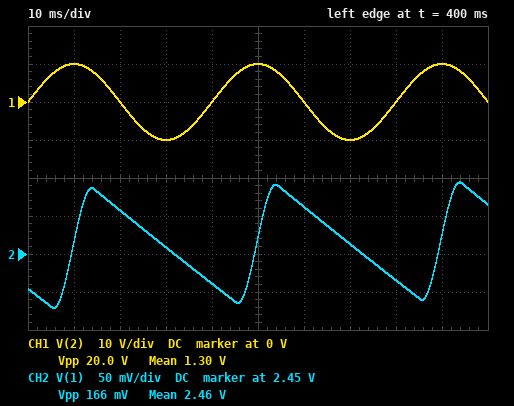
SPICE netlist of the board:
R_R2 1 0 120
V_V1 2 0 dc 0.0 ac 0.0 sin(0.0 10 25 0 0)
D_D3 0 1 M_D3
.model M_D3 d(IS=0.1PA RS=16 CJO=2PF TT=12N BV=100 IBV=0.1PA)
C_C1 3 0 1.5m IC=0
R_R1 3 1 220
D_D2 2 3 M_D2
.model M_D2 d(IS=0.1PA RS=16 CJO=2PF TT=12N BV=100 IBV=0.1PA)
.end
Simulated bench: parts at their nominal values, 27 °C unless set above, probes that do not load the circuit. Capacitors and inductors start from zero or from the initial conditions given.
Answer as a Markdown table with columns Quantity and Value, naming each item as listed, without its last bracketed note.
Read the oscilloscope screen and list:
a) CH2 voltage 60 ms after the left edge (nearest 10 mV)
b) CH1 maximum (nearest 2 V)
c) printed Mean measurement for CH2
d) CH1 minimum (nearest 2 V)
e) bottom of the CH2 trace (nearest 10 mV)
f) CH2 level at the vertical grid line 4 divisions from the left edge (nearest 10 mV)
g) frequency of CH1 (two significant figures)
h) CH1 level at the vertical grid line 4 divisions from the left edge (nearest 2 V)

| Quantity | Value |
|---|---|
| CH2 voltage 60 ms after the left edge | 2.51 V |
| CH1 maximum | 10 V |
| printed Mean measurement for CH2 | 2.46 V |
| CH1 minimum | -10 V |
| bottom of the CH2 trace | 2.38 V |
| CH2 level at the vertical grid line 4 divisions from the left edge | 2.41 V |
| frequency of CH1 | 25 Hz |
| CH1 level at the vertical grid line 4 divisions from the left edge | 0 V |
